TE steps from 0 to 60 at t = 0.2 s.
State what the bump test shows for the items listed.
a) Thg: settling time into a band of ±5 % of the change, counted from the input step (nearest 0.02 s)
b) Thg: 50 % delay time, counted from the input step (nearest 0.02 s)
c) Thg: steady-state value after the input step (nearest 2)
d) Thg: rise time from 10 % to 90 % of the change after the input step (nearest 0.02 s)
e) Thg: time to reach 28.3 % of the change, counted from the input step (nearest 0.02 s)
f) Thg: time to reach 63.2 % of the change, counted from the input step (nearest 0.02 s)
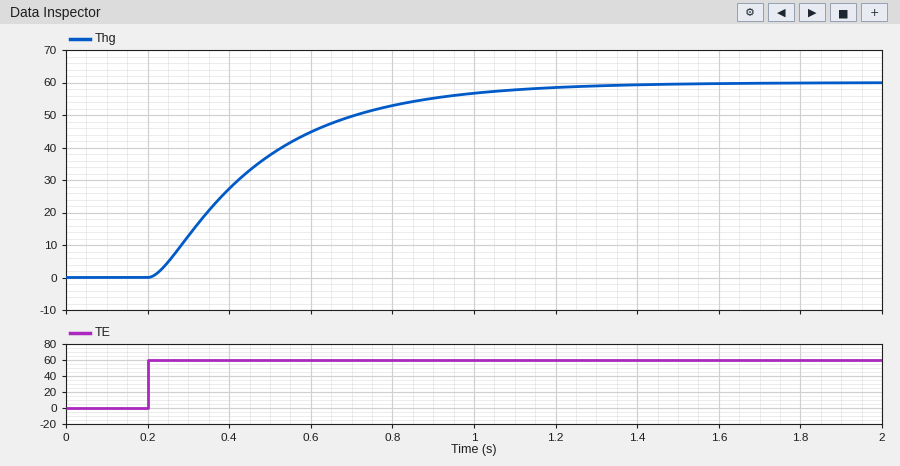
0.82 s
0.22 s
60
0.58 s
0.12 s
0.30 s
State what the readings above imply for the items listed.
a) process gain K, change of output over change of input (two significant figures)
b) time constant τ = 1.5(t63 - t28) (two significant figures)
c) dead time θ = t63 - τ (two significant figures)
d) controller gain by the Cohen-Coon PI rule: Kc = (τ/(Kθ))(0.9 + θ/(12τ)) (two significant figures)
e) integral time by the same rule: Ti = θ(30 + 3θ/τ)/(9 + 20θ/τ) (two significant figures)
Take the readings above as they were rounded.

1.0
0.27 s
0.030 s
8.2
0.081 s
